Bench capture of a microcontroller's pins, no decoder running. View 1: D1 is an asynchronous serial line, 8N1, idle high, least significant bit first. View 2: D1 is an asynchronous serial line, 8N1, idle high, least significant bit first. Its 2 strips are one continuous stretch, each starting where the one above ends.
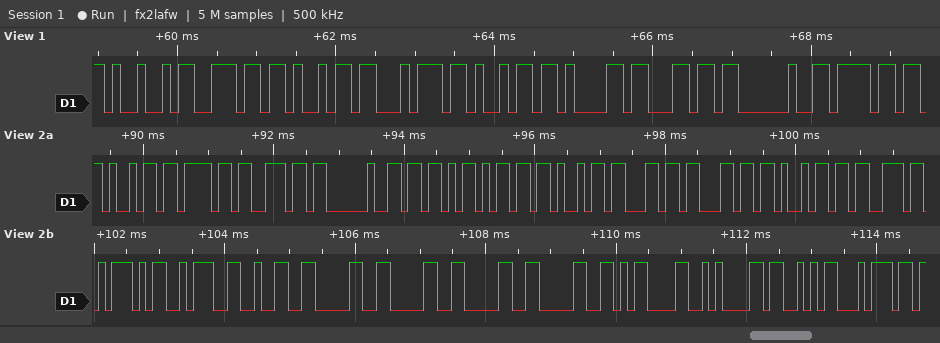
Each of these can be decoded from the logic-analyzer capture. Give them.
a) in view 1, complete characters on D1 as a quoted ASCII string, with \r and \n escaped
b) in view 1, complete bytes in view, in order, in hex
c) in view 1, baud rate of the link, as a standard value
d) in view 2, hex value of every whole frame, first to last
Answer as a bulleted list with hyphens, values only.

- "Initial o"
- 0x49 0x6E 0x69 0x74 0x69 0x61 0x6C 0x20 0x6F
- 9600 baud
- 69 6F 6E 20 5B 6D 69 6C 6C 69 73 5D 3A 32 30 30 30 30 0D 0A 53 74
